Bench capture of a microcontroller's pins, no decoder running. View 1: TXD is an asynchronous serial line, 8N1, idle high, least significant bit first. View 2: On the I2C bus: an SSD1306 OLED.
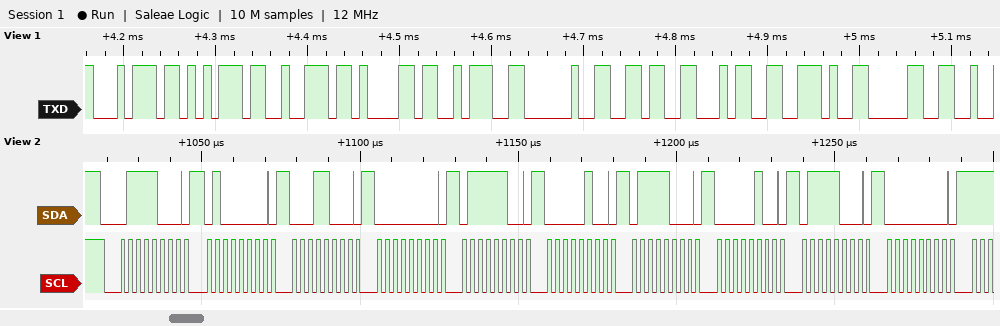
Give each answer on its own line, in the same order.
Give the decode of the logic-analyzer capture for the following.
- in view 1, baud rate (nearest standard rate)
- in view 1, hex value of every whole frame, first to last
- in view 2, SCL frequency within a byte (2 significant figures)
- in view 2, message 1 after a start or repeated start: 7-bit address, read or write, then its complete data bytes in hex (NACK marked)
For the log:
115200 baud
74 75 72 61 3A 20 36 34 2E 30
400 kHz
0x3C write: 40 18 00 7C 04 78 04 78 00
